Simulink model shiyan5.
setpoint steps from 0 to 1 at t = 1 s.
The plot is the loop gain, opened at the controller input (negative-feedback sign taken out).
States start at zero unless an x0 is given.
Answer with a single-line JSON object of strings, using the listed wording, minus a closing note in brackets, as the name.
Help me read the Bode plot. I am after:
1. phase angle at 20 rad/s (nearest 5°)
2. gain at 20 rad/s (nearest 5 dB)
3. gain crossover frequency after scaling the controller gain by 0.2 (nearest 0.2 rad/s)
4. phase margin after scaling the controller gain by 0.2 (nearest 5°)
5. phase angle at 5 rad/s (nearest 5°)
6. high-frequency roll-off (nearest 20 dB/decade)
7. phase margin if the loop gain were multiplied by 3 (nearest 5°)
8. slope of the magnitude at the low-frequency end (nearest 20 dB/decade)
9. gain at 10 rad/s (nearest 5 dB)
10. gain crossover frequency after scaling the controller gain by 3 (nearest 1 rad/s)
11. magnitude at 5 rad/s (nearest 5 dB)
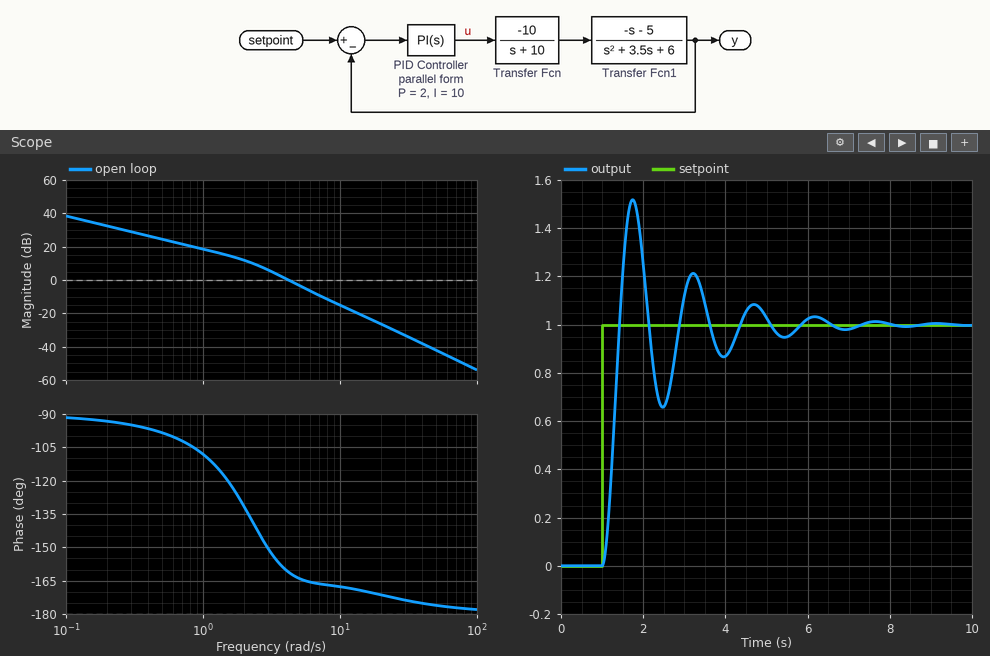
{"phase angle at 20 rad/s": "-170°", "gain at 20 rad/s": "-25 dB", "gain crossover frequency after scaling the controller gain by 0.2": "1.6 rad/s", "phase margin after scaling the controller gain by 0.2": "55°", "phase angle at 5 rad/s": "-165°", "high-frequency roll-off": "-40 dB/decade", "phase margin if the loop gain were multiplied by 3": "15°", "slope of the magnitude at the low-frequency end": "-20 dB/decade", "gain at 10 rad/s": "-15 dB", "gain crossover frequency after scaling the controller gain by 3": "7 rad/s", "magnitude at 5 rad/s": "-5 dB"}
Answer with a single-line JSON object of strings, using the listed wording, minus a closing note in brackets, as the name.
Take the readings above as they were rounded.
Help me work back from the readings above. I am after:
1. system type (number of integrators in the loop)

{"system type": "1"}
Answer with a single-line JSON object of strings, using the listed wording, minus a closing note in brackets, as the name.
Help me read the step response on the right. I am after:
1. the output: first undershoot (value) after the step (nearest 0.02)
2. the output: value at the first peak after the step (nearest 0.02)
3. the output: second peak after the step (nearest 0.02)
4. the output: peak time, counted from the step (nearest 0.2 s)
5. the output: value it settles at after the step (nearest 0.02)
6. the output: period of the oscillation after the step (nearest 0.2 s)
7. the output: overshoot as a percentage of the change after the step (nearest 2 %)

{"the output: first undershoot (value) after the step": "0.66", "the output: value at the first peak after the step": "1.52", "the output: second peak after the step": "1.22", "the output: peak time, counted from the step": "0.8 s", "the output: value it settles at after the step": "1.00", "the output: period of the oscillation after the step": "1.4 s", "the output: overshoot as a percentage of the change after the step": "52 %"}
